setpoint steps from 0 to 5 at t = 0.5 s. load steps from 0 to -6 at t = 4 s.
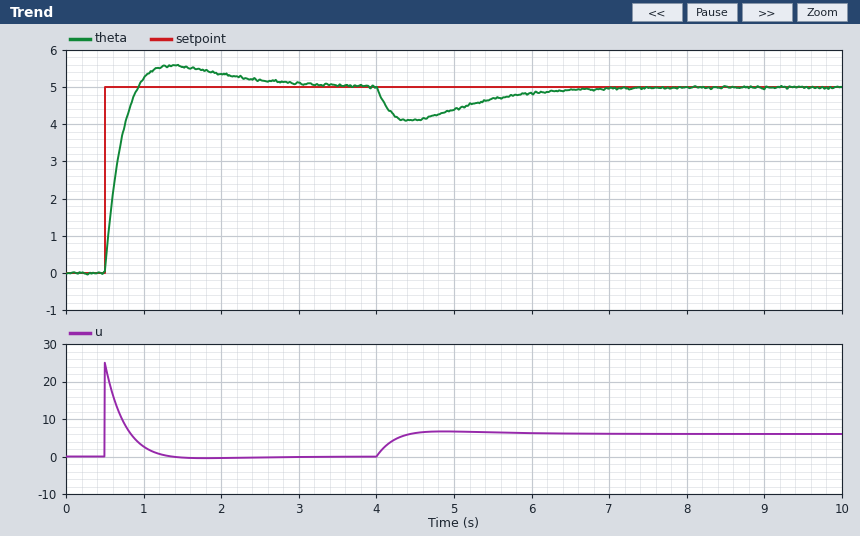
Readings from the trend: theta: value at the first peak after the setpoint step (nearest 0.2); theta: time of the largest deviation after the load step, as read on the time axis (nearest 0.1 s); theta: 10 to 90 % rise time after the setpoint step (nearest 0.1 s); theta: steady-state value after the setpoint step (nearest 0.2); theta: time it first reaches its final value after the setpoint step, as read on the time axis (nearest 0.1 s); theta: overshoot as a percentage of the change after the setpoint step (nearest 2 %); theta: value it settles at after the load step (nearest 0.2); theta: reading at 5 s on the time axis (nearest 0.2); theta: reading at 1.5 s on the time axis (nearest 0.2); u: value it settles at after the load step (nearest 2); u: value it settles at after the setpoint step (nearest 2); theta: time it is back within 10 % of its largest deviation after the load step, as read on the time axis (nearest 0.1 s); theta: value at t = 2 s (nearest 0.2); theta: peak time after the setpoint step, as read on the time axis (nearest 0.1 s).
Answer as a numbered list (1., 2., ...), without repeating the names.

1. 5.6
2. 4.4 s
3. 0.3 s
4. 5.0
5. 0.9 s
6. 12 %
7. 5.0
8. 4.4
9. 5.6
10. 6
11. 0
12. 6.4 s
13. 5.4
14. 1.4 s
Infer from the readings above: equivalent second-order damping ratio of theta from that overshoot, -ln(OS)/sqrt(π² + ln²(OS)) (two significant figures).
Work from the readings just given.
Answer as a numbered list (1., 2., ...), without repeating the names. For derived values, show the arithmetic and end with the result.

1. ln(0.12) = -2.120; 2.120 / sqrt(9.870 + 4.496) = 0.56
